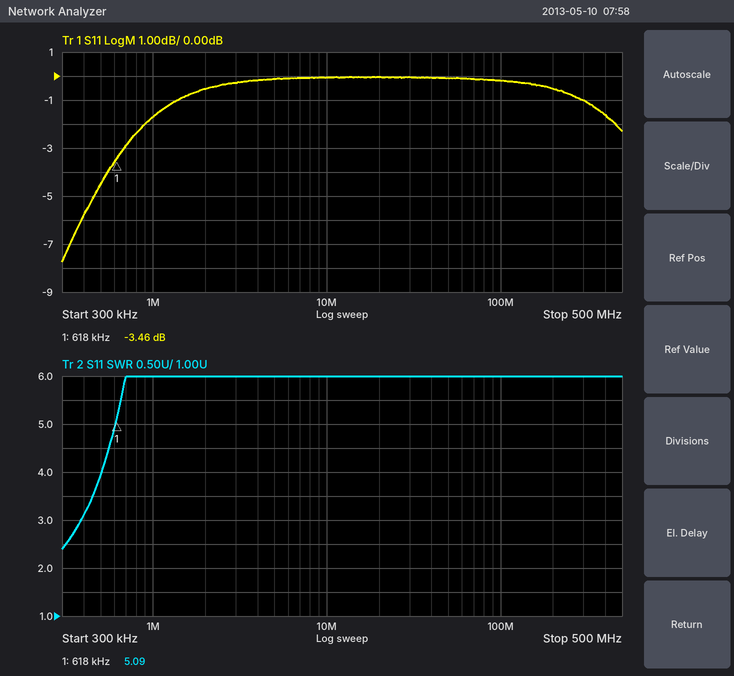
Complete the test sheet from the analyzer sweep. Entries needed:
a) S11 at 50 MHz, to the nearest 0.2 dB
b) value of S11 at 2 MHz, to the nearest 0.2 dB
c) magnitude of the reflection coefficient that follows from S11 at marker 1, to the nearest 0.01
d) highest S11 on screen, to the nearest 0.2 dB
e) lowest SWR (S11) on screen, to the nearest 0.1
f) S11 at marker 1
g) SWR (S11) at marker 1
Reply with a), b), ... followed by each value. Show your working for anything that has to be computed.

a) 0.0 dB
b) -0.6 dB
c) 10^(-3.46/20) ≈ 0.67
d) 0.0 dB
e) 2.4
f) -3.46 dB
g) 5.09
